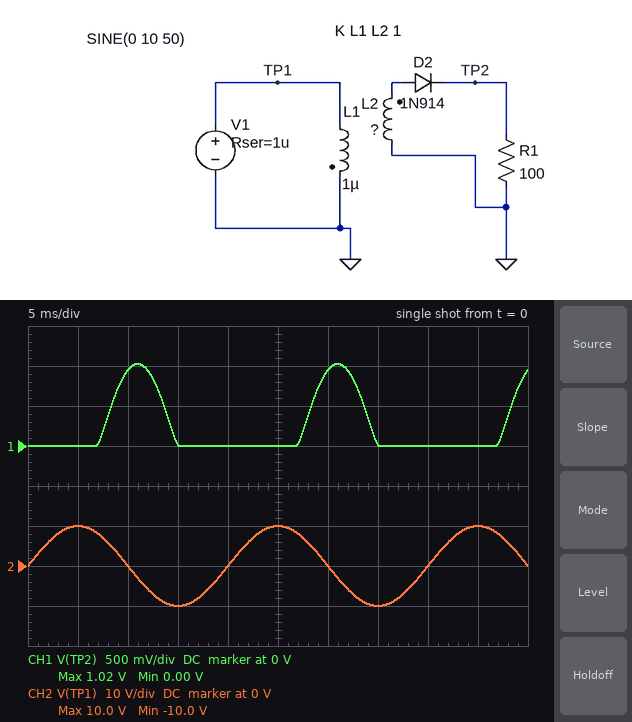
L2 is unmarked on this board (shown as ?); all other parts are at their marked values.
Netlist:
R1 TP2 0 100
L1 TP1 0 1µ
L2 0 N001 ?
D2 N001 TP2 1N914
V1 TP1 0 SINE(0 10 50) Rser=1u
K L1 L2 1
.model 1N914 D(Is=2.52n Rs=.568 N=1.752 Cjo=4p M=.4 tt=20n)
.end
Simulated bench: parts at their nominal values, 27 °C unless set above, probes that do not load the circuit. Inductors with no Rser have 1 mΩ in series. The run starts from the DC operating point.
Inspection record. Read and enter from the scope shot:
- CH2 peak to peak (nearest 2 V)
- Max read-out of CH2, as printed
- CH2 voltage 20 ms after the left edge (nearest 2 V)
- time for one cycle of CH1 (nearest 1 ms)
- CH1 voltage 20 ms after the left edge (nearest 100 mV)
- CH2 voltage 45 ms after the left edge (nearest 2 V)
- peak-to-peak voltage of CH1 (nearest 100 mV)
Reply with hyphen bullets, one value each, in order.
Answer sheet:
- 20 V
- 10.0 V
- 0 V
- 20 ms
- 0 V
- 10 V
- 1.0 V
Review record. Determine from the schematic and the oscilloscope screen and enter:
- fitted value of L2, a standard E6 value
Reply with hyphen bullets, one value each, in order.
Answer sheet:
- 330 nH
